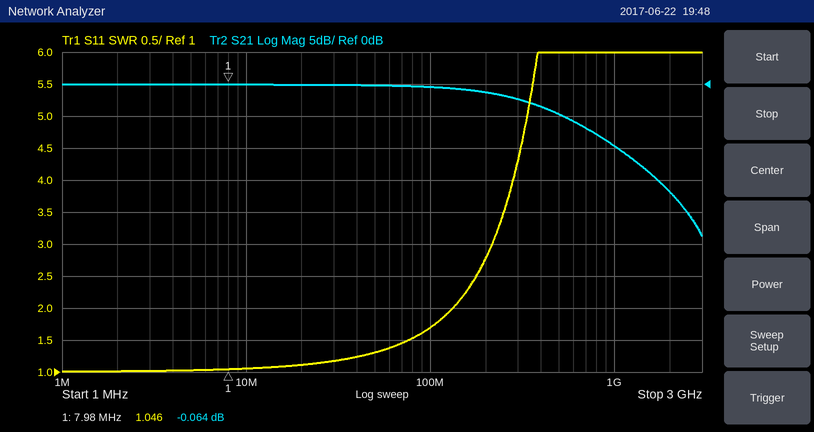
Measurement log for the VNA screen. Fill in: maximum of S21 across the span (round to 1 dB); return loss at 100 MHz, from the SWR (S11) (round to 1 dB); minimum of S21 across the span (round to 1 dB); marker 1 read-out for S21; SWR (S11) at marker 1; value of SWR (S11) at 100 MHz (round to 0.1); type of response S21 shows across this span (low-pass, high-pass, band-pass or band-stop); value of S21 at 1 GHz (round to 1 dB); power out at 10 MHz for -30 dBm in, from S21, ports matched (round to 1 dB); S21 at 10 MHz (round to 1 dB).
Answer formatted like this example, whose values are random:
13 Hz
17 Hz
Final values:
0 dB
12 dB
-24 dB
-0.064 dB
1.046
1.7
low-pass
-10 dB
-30 dBm
0 dB
